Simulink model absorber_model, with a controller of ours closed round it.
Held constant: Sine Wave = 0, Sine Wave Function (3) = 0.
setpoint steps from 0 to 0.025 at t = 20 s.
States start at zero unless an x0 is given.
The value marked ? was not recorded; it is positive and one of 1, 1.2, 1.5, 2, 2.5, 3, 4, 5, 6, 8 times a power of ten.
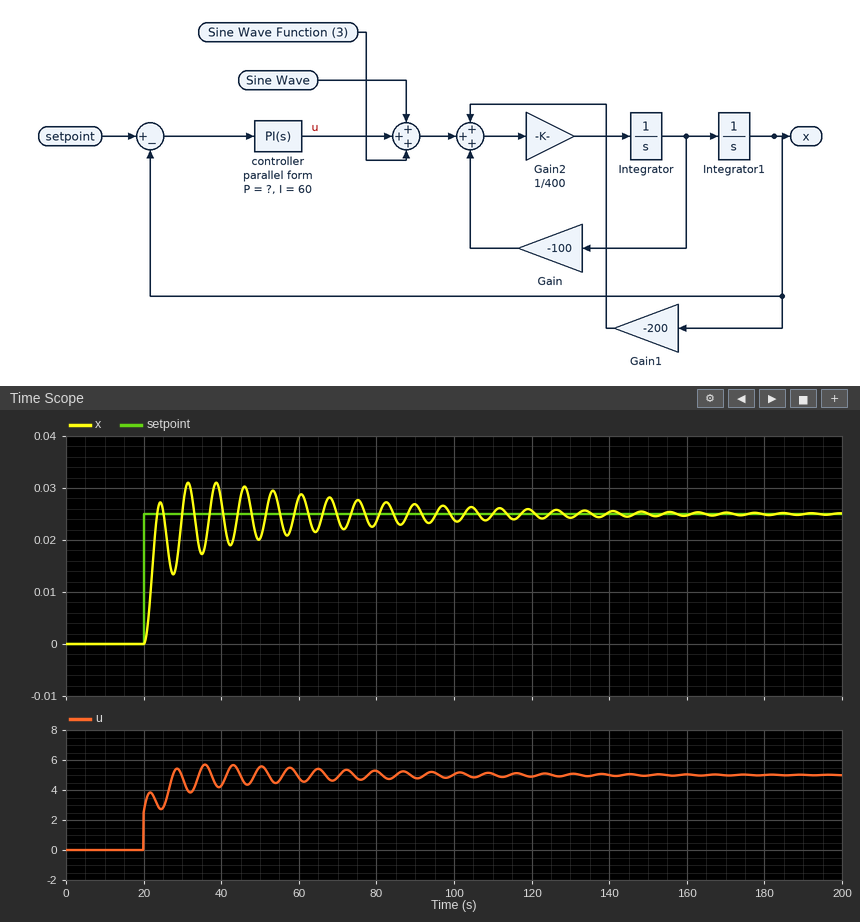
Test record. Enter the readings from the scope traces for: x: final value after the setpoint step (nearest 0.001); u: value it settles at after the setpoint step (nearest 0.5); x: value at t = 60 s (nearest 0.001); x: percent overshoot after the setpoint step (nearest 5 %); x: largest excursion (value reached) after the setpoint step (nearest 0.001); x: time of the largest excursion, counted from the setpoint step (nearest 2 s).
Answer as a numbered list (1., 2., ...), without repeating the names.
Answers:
1. 0.025
2. 5.0
3. 0.028
4. 25 %
5. 0.031
6. 18 s
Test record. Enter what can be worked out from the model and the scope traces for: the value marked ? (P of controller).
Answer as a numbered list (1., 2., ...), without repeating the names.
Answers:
1. 100
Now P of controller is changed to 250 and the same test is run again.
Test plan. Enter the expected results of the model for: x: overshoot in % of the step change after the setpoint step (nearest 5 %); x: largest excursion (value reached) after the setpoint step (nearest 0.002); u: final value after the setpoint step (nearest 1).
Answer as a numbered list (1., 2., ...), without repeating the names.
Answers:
1. 20 %
2. 0.030
3. 5
